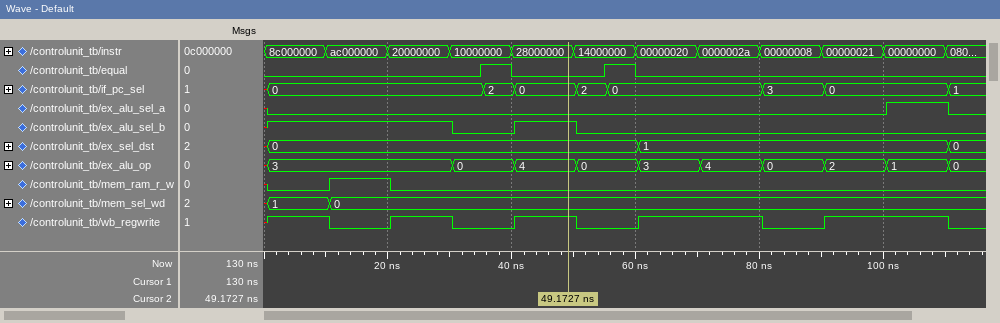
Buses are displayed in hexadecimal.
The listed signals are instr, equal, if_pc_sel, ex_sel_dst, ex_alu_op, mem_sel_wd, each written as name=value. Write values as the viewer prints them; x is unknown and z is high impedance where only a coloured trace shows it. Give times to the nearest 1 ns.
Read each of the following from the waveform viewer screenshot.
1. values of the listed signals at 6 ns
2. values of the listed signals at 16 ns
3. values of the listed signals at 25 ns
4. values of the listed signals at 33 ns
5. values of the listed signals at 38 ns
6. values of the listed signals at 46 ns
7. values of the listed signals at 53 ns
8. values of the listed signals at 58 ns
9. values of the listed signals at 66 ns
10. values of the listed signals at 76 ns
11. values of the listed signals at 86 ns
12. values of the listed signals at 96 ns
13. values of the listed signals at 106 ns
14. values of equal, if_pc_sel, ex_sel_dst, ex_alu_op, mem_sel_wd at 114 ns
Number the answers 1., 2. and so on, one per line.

1. instr=8c000000, equal=0, if_pc_sel=0, ex_sel_dst=0, ex_alu_op=3, mem_sel_wd=1
2. instr=ac000000, equal=0, if_pc_sel=0, ex_sel_dst=0, ex_alu_op=3, mem_sel_wd=0
3. instr=20000000, equal=0, if_pc_sel=0, ex_sel_dst=0, ex_alu_op=3, mem_sel_wd=0
4. instr=10000000, equal=0, if_pc_sel=0, ex_sel_dst=0, ex_alu_op=0, mem_sel_wd=0
5. instr=10000000, equal=1, if_pc_sel=2, ex_sel_dst=0, ex_alu_op=0, mem_sel_wd=0
6. instr=28000000, equal=0, if_pc_sel=0, ex_sel_dst=0, ex_alu_op=4, mem_sel_wd=0
7. instr=14000000, equal=0, if_pc_sel=2, ex_sel_dst=0, ex_alu_op=0, mem_sel_wd=0
8. instr=14000000, equal=1, if_pc_sel=0, ex_sel_dst=0, ex_alu_op=0, mem_sel_wd=0
9. instr=00000020, equal=0, if_pc_sel=0, ex_sel_dst=1, ex_alu_op=3, mem_sel_wd=0
10. instr=0000002a, equal=0, if_pc_sel=0, ex_sel_dst=1, ex_alu_op=4, mem_sel_wd=0
11. instr=00000008, equal=0, if_pc_sel=3, ex_sel_dst=1, ex_alu_op=0, mem_sel_wd=0
12. instr=00000021, equal=0, if_pc_sel=0, ex_sel_dst=1, ex_alu_op=2, mem_sel_wd=0
13. instr=00000000, equal=0, if_pc_sel=0, ex_sel_dst=1, ex_alu_op=1, mem_sel_wd=0
14. equal=0, if_pc_sel=1, ex_sel_dst=0, ex_alu_op=0, mem_sel_wd=0
